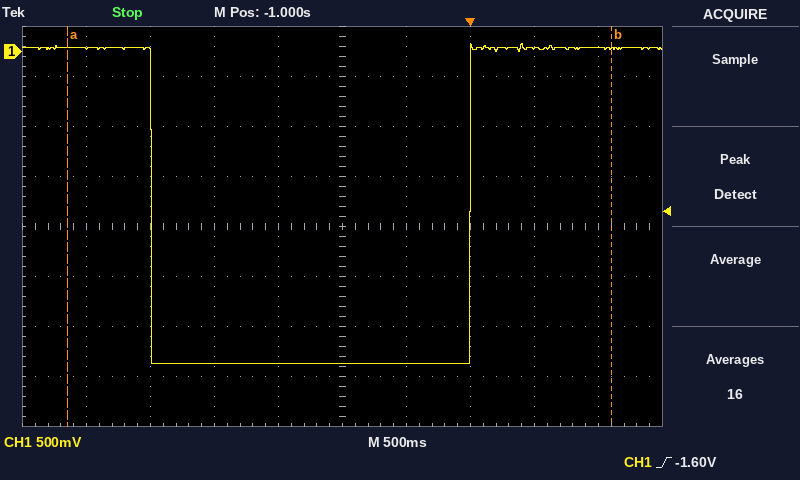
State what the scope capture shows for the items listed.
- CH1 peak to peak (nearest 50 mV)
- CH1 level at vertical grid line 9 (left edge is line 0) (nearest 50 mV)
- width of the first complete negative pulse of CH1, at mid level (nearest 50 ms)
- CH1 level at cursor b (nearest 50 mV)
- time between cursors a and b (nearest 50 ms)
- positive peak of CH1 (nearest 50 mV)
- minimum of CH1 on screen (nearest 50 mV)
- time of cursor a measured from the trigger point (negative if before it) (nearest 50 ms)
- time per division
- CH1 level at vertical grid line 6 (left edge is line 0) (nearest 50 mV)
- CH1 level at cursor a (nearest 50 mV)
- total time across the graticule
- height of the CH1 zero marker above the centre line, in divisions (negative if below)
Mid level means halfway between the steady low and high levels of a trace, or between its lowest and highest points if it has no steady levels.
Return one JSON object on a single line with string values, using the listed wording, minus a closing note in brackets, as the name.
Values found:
{"CH1 peak to peak": "3.20 V", "CH1 level at vertical grid line 9 (left edge is line 0)": "50 mV", "width of the first complete negative pulse of CH1, at mid level": "2.50 s", "CH1 level at cursor b": "50 mV", "time between cursors a and b": "4.25 s", "positive peak of CH1": "100 mV", "minimum of CH1 on screen": "-3.10 V", "time of cursor a measured from the trigger point (negative if before it)": "-3.15 s", "time per division": "500 ms", "CH1 level at vertical grid line 6 (left edge is line 0)": "-3.10 V", "CH1 level at cursor a": "50 mV", "total time across the graticule": "5 s", "height of the CH1 zero marker above the centre line, in divisions": "+3.5 div"}
